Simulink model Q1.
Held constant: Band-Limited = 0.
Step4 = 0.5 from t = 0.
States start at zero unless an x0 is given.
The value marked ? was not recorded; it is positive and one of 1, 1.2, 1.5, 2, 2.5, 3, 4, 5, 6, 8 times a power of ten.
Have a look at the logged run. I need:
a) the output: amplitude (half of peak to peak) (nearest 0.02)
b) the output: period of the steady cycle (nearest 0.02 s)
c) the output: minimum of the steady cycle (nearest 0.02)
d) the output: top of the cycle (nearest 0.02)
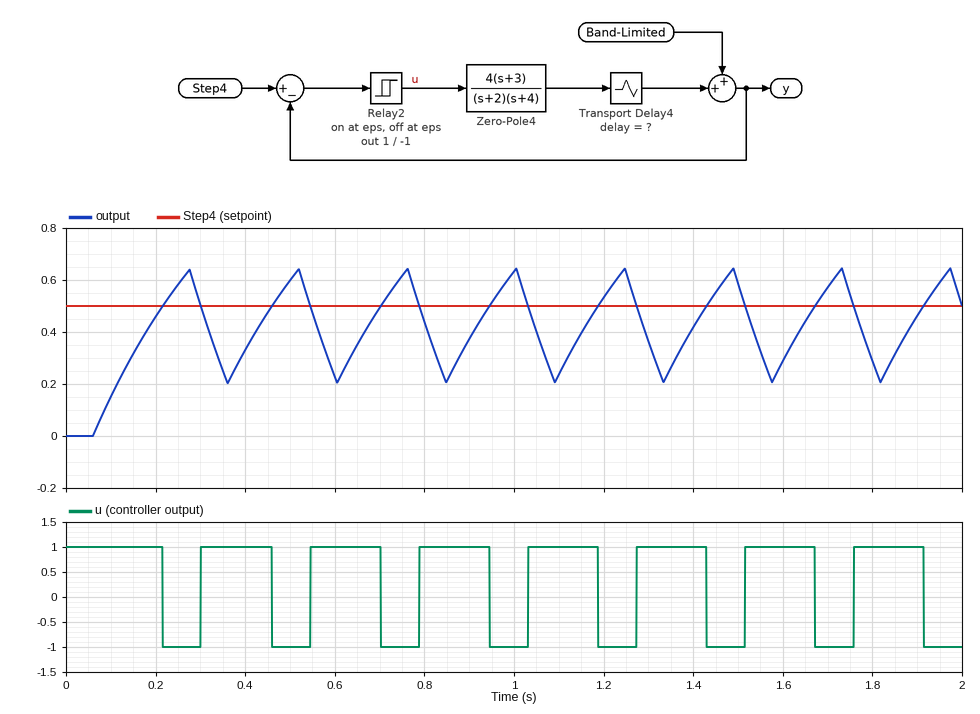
0.22
0.24 s
0.20
0.64
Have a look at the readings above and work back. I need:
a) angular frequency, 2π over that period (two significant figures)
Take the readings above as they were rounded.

26 rad/s
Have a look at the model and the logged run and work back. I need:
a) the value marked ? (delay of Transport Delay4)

0.06
